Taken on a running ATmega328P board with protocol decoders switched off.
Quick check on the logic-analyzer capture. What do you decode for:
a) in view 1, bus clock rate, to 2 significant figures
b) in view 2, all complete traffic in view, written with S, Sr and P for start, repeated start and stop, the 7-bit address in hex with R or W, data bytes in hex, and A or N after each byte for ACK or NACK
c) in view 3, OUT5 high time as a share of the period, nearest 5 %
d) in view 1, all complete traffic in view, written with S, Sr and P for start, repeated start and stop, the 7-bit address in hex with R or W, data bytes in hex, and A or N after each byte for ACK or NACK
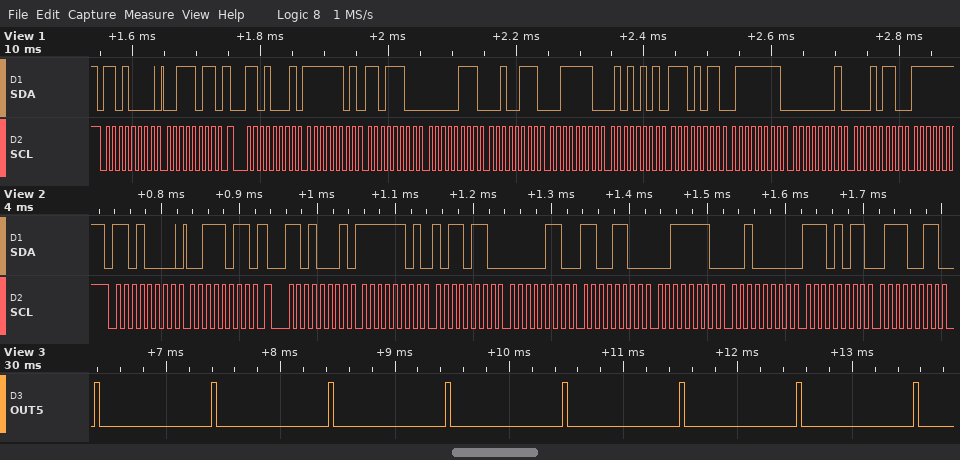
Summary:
100 kHz
S 68W A 3B A Sr 68R A FD A B6 A 06 A CC A 3E A 20 A EB A 73 A
5 %
S 68W A 3B A Sr 68R A FD A DC A 07 A 27 A 3E A 55 A EB A 7F A 01 A 16 A
